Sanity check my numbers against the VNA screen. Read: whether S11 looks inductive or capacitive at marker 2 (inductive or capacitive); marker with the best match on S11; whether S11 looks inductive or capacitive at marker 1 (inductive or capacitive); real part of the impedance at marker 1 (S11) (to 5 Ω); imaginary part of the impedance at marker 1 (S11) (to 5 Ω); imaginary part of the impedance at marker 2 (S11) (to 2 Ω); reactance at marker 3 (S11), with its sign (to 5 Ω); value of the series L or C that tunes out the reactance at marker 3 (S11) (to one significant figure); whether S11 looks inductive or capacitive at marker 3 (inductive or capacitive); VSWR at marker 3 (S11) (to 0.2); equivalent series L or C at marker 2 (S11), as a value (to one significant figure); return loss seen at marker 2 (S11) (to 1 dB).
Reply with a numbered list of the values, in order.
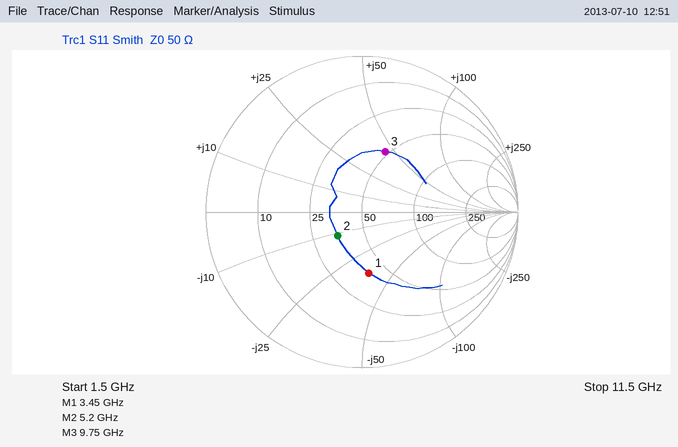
1. capacitive
2. marker 2
3. capacitive
4. 40 Ω
5. -35 Ω
6. -12 Ω
7. +45 Ω
8. 400 fF
9. inductive
10. 2.4
11. 3 pF
12. 13 dB
